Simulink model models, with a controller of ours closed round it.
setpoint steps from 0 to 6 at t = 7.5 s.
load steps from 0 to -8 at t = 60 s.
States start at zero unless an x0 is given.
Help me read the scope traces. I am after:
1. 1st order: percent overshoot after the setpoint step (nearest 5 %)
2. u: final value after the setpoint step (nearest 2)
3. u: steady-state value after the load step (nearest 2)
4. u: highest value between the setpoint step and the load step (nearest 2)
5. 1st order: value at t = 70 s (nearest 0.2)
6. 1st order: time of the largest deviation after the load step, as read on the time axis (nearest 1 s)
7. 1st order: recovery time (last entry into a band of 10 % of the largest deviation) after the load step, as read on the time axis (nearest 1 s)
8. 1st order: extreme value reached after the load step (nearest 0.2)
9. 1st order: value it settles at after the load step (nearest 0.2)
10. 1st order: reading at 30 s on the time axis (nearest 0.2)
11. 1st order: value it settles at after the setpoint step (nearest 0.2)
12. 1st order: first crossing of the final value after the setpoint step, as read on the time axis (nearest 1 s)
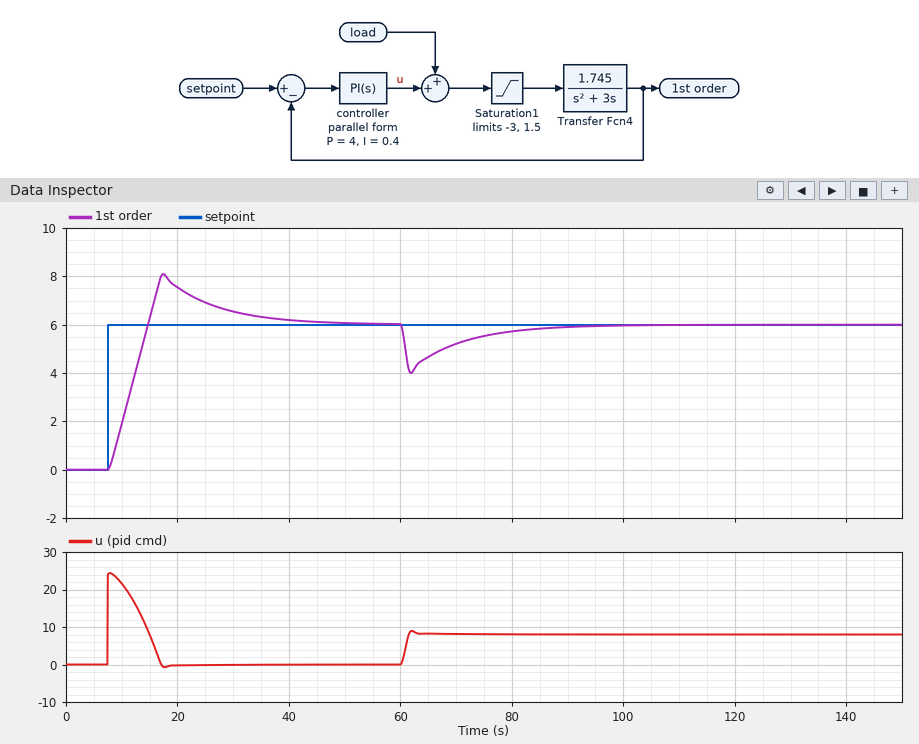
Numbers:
35 %
0
8
24
5.2
62 s
83 s
4.0
6.0
6.6
6.0
15 s
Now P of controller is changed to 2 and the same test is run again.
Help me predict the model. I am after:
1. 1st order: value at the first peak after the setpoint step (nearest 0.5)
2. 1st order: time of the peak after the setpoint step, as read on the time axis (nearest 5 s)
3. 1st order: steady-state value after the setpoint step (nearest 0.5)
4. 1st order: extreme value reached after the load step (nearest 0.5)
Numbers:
9.5
20 s
6.0
2.5
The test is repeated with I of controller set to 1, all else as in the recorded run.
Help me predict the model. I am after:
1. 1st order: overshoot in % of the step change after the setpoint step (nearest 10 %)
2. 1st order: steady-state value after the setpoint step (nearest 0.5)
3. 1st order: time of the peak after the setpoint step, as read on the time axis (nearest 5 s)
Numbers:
60 %
6.0
20 s
